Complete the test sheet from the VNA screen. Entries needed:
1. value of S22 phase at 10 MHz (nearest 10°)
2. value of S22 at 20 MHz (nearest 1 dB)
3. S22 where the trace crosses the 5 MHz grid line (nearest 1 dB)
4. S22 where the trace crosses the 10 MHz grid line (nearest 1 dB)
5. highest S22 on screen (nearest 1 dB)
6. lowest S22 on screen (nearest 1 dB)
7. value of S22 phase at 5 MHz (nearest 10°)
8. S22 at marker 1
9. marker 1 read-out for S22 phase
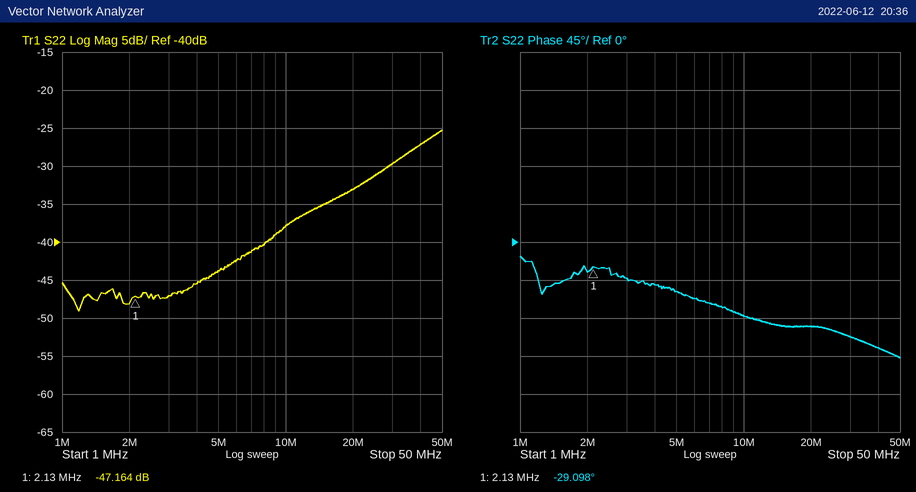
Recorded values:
-90°
-33 dB
-44 dB
-38 dB
-25 dB
-49 dB
-60°
-47.164 dB
-29.098°
